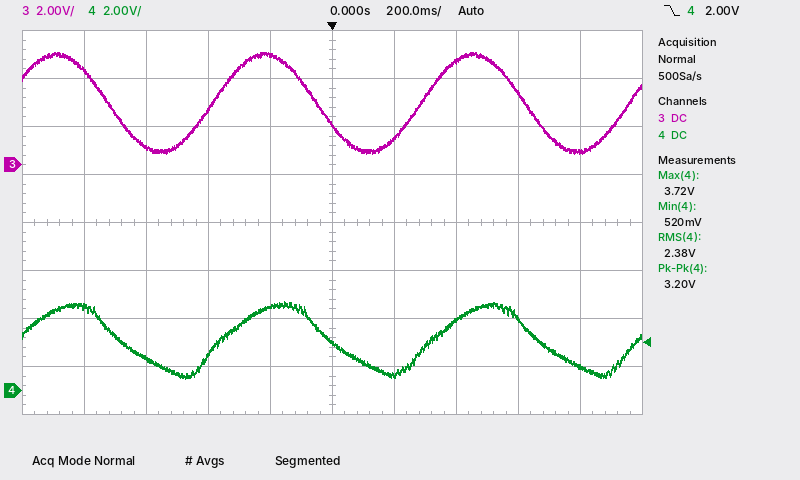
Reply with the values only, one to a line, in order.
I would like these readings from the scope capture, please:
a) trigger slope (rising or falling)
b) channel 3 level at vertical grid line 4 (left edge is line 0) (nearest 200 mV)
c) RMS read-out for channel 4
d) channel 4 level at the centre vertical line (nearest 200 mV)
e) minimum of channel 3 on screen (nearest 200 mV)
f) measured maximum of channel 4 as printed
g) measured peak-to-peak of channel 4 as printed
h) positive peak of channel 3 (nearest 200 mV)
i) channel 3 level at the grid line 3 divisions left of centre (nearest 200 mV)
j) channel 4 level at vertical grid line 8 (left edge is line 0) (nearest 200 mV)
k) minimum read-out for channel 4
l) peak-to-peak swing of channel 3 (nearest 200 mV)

falling
4.6 V
2.38 V
2.0 V
400 mV
3.72 V
3.20 V
4.6 V
800 mV
3.0 V
520 mV
4.2 V
